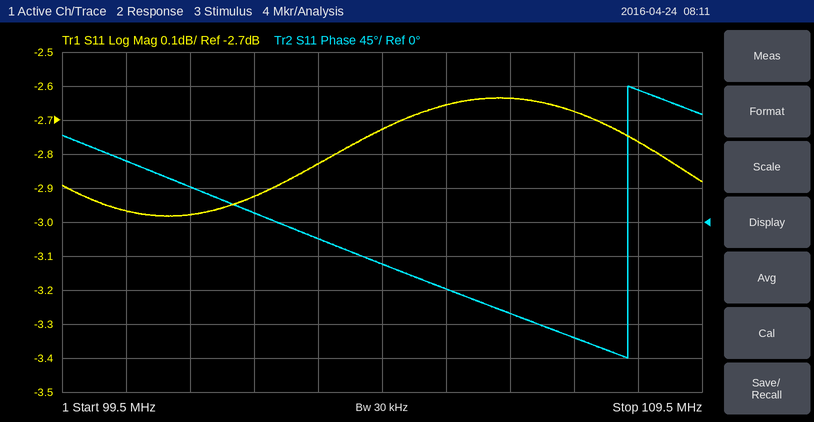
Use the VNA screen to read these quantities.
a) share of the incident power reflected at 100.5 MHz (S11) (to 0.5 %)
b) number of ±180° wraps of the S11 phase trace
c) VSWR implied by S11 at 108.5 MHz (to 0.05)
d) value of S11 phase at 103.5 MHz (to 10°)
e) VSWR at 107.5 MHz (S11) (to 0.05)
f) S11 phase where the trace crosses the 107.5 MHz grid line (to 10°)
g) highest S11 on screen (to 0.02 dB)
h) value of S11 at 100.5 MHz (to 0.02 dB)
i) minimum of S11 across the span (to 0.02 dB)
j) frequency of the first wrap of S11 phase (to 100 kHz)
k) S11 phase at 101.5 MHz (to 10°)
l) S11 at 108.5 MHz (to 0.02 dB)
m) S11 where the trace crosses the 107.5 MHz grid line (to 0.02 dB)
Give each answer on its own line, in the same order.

50.5 %
1
6.35
-20°
6.55
-150°
-2.64 dB
-2.96 dB
-2.98 dB
108.3 MHz
50°
-2.76 dB
-2.68 dB
